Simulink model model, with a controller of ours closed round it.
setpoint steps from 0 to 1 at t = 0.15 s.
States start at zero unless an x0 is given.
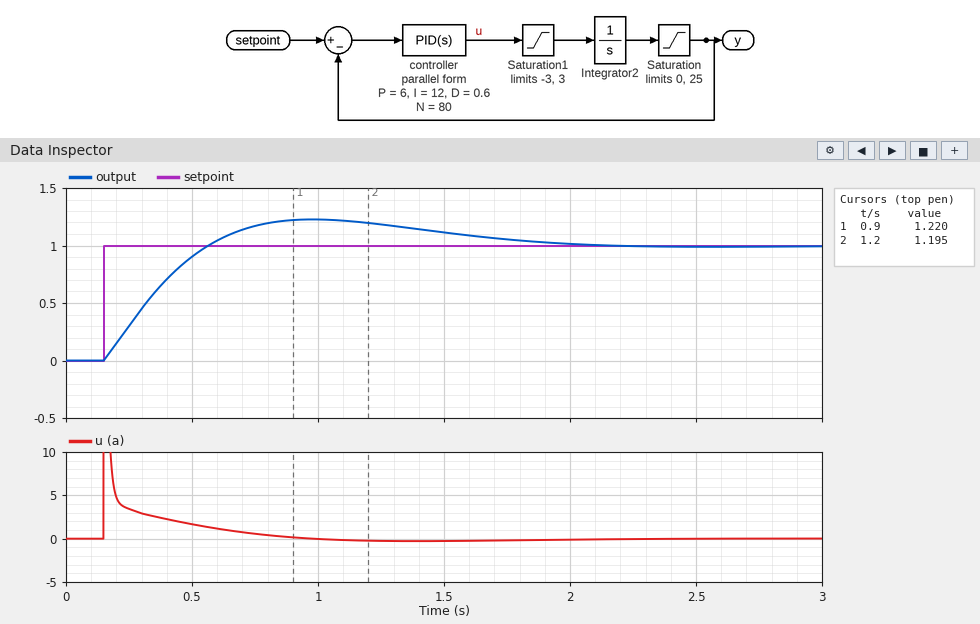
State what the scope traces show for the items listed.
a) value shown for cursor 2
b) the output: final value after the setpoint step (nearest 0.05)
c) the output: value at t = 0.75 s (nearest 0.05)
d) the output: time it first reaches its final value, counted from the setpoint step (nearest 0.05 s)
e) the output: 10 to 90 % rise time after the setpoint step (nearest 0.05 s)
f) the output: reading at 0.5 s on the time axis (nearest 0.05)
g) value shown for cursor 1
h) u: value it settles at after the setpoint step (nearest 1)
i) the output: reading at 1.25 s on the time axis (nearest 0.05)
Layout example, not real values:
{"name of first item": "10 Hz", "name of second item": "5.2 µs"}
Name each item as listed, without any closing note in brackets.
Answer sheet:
{"value shown for cursor 2": "1.195", "the output: final value after the setpoint step": "1.00", "the output: value at t = 0.75 s": "1.15", "the output: time it first reaches its final value, counted from the setpoint step": "0.40 s", "the output: 10 to 90 % rise time after the setpoint step": "0.30 s", "the output: reading at 0.5 s on the time axis": "0.90", "value shown for cursor 1": "1.220", "u: value it settles at after the setpoint step": "0", "the output: reading at 1.25 s on the time axis": "1.20"}
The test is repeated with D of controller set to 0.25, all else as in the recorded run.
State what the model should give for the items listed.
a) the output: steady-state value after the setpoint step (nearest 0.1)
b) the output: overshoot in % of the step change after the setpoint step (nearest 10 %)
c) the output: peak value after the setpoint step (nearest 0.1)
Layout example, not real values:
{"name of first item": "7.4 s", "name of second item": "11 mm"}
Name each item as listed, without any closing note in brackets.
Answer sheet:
{"the output: steady-state value after the setpoint step": "1.0", "the output: overshoot in % of the step change after the setpoint step": "20 %", "the output: peak value after the setpoint step": "1.2"}
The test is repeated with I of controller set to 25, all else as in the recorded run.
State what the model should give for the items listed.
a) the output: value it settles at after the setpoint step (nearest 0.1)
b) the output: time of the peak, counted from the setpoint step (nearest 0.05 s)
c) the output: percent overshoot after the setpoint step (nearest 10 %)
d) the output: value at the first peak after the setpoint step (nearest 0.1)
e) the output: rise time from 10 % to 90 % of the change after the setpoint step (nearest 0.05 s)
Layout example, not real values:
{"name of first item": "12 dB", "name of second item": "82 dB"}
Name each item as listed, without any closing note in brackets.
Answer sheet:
{"the output: value it settles at after the setpoint step": "1.0", "the output: time of the peak, counted from the setpoint step": "0.65 s", "the output: percent overshoot after the setpoint step": "40 %", "the output: value at the first peak after the setpoint step": "1.4", "the output: rise time from 10 % to 90 % of the change after the setpoint step": "0.25 s"}
